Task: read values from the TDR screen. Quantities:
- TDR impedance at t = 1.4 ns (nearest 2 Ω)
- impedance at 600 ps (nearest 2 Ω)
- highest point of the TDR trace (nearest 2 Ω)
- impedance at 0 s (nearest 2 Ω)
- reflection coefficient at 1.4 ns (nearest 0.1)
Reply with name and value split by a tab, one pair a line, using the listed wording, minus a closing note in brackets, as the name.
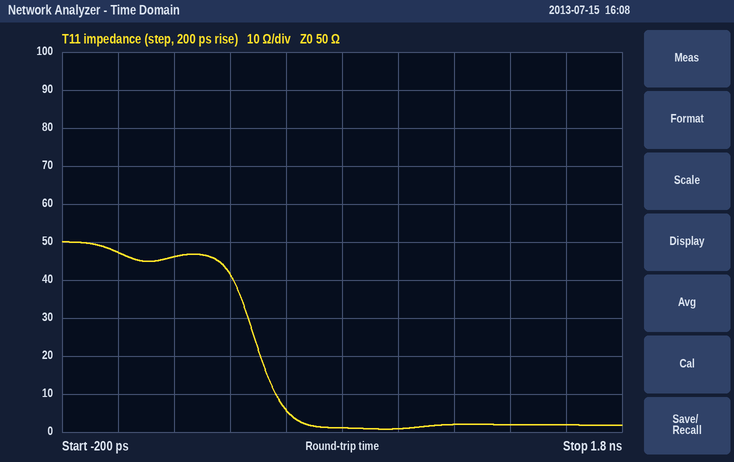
TDR impedance at t = 1.4 ns	2 Ω
impedance at 600 ps	6 Ω
highest point of the TDR trace	50 Ω
impedance at 0 s	48 Ω
reflection coefficient at 1.4 ns	-0.9
